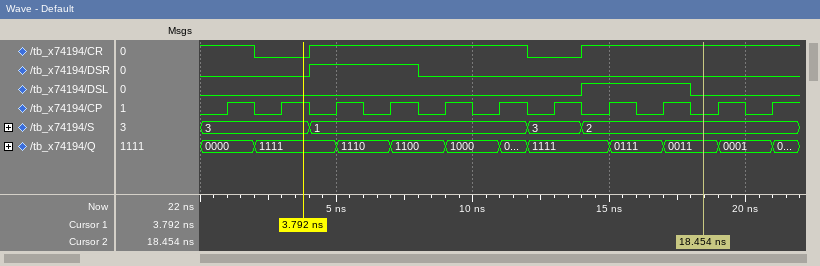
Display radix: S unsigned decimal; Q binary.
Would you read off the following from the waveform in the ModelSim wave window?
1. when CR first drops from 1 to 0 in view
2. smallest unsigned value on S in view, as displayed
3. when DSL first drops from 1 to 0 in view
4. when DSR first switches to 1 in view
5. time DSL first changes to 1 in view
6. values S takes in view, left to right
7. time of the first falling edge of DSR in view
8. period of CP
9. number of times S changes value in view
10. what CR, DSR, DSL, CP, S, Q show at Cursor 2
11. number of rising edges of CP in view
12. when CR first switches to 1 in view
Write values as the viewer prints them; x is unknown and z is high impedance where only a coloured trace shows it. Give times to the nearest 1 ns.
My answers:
2 ns
1
18 ns
4 ns
14 ns
3, 1, 3, 2
8 ns
2 ns
3
CR=1, DSR=0, DSL=0, CP=0, S=2, Q=0011
11
4 ns
